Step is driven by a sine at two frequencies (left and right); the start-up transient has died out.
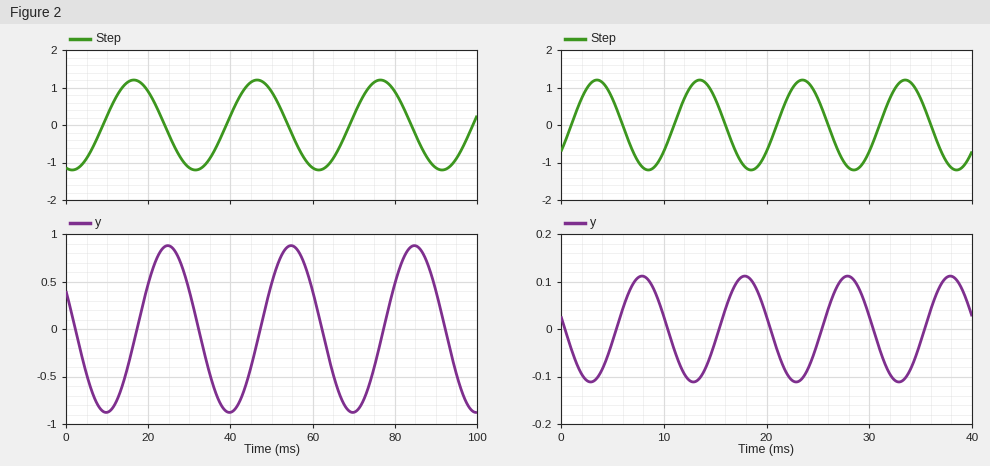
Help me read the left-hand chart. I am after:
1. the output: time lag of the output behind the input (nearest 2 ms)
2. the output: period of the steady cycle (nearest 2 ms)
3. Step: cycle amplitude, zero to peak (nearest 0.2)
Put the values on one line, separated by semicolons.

8 ms; 30 ms; 1.2
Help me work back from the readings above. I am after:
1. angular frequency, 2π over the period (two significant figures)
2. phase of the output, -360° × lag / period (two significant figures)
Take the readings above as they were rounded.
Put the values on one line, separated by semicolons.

0.21 rad/ms; -96°
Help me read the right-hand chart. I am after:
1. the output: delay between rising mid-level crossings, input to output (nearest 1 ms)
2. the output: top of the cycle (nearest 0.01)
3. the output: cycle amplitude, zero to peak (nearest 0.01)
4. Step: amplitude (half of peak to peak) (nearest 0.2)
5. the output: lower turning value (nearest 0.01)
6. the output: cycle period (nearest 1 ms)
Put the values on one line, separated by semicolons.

4 ms; 0.11; 0.11; 1.2; -0.11; 10 ms
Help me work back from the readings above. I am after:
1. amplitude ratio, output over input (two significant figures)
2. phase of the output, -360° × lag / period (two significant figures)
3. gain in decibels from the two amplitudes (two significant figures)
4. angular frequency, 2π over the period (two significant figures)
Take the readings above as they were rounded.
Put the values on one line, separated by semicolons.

0.092; -140°; -21 dB; 0.63 rad/ms
